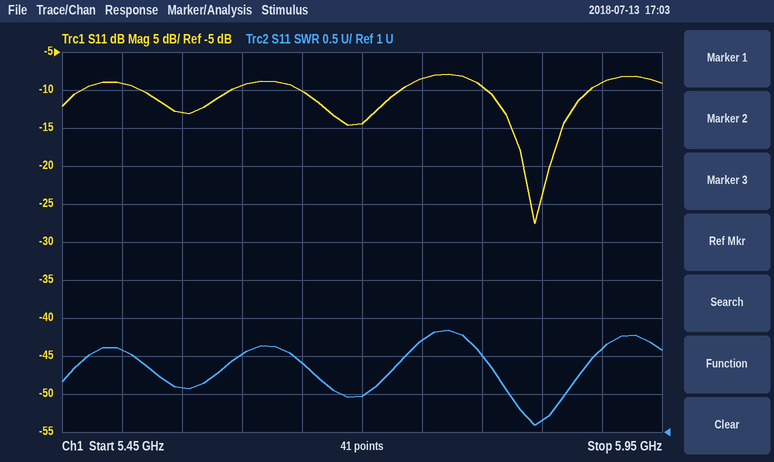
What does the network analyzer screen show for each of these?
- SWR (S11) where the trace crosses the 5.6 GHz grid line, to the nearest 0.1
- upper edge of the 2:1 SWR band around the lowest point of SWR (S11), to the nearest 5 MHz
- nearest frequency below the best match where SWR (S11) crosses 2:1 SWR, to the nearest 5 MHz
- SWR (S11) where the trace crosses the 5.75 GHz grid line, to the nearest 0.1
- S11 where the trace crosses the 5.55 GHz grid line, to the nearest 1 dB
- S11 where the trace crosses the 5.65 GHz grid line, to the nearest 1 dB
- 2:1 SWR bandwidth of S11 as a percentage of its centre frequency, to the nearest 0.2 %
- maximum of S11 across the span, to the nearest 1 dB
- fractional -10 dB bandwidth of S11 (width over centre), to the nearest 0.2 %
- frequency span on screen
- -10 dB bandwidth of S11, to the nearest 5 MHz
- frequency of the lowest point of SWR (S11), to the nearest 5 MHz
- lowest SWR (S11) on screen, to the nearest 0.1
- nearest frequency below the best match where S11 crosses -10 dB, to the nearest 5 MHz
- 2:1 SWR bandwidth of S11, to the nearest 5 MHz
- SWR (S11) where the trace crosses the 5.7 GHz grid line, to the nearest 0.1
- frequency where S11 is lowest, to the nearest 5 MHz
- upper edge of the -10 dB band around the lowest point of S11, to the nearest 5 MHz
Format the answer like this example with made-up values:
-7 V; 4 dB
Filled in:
2.0; 5.895 GHz; 5.800 GHz; 2.2; -13 dB; -10 dB; 1.6 %; -8 dB; 1.4 %; 500 MHz; 85 MHz; 5.845 GHz; 1.1; 5.805 GHz; 95 MHz; 1.5; 5.845 GHz; 5.890 GHz
